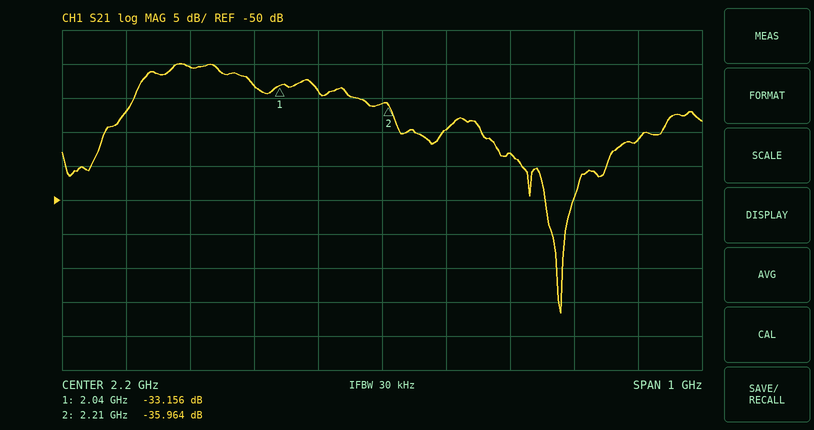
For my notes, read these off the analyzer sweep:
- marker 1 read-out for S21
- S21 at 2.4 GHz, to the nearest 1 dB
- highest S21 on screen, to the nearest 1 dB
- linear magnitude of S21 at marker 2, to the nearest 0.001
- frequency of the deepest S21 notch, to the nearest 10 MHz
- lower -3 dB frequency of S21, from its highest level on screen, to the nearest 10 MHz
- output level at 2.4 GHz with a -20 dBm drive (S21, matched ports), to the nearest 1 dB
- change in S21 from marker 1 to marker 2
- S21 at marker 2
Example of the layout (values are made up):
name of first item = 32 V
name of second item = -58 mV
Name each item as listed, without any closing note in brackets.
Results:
marker 1 read-out for S21 = -33.156 dB
S21 at 2.4 GHz, to the nearest 1 dB = -43 dB
highest S21 on screen, to the nearest 1 dB = -30 dB
linear magnitude of S21 at marker 2, to the nearest 0.001 = 0.016
frequency of the deepest S21 notch, to the nearest 10 MHz = 2.48 GHz
lower -3 dB frequency of S21, from its highest level on screen, to the nearest 10 MHz = 1.82 GHz
output level at 2.4 GHz with a -20 dBm drive (S21, matched ports), to the nearest 1 dB = -63 dBm
change in S21 from marker 1 to marker 2 = -2.808 dB
S21 at marker 2 = -35.964 dB
